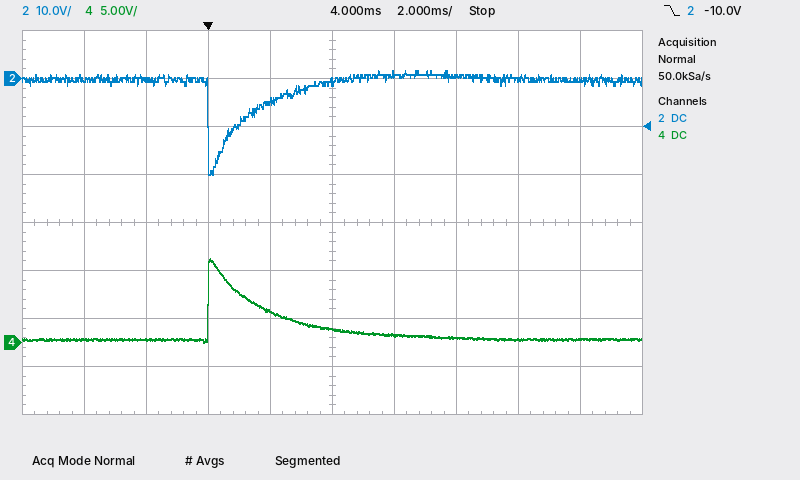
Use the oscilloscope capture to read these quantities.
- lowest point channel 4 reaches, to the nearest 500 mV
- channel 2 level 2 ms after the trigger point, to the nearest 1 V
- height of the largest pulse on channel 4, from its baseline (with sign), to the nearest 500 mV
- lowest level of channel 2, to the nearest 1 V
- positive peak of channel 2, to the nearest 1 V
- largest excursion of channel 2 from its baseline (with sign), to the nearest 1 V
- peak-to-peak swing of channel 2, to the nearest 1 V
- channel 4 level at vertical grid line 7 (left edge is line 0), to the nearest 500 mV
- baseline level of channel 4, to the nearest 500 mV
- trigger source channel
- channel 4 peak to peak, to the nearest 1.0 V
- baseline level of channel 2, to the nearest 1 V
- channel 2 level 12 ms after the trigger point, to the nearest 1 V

0.0 V
-5 V
+8.5 V
-20 V
2 V
-20 V
22 V
500 mV
500 mV
channel 2
9.0 V
0 V
0 V
